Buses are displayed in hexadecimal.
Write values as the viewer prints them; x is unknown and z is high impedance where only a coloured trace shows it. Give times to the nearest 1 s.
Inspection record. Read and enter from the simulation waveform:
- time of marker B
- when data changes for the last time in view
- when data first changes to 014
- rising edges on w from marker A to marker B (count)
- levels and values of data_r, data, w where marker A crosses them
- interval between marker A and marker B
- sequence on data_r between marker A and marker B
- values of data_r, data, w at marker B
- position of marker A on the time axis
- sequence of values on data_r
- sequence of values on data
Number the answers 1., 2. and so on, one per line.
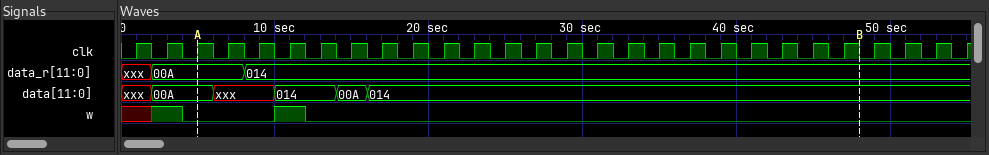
1. 48 s
2. 16 s
3. 10 s
4. 1
5. data_r=00A, data=00A, w=0
6. 43 s
7. 00A, 014
8. data_r=014, data=014, w=0
9. 5 s
10. xxx, 00A, 014
11. xxx, 00A, xxx, 014, 00A, 014
